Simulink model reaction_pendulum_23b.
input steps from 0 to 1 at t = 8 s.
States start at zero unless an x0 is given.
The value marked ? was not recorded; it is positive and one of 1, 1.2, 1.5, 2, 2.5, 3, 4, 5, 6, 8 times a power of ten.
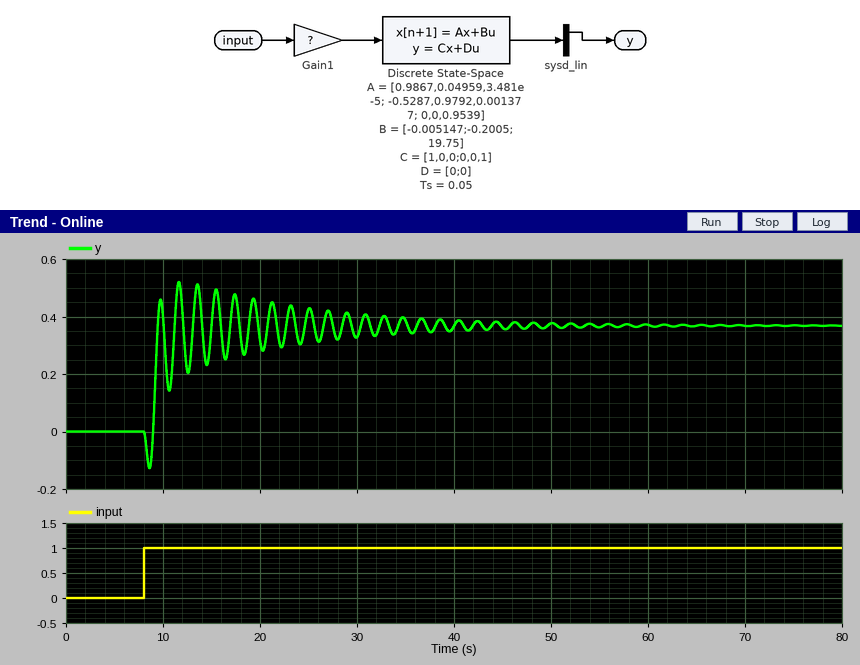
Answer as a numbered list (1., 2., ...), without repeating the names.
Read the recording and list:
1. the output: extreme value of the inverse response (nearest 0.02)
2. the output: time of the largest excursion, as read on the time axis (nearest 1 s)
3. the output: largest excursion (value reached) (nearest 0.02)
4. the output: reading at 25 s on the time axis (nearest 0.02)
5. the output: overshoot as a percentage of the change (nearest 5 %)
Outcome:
1. -0.12
2. 12 s
3. 0.52
4. 0.42
5. 40 %
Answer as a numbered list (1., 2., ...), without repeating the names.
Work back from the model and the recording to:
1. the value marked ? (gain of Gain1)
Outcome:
1. 0.5
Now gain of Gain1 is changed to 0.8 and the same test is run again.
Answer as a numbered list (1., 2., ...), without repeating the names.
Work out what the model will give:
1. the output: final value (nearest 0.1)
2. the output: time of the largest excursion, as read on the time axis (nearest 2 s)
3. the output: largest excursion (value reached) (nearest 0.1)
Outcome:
1. 0.6
2. 12 s
3. 0.8
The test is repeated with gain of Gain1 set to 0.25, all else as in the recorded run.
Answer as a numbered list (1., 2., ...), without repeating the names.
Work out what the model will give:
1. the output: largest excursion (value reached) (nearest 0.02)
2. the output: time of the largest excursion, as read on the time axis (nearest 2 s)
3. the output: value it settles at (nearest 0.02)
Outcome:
1. 0.26
2. 12 s
3. 0.18
